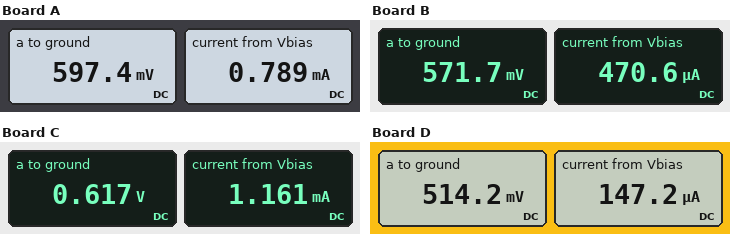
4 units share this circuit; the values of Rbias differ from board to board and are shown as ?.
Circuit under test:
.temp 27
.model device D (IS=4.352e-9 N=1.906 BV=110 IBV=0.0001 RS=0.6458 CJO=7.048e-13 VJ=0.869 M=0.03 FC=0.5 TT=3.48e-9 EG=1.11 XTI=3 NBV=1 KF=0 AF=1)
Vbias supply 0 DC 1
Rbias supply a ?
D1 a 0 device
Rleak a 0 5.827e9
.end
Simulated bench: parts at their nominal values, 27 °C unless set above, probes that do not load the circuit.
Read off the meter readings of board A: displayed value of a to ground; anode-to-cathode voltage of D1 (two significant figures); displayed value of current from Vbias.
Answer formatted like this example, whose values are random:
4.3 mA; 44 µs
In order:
597.4 mV; 600 mV; 0.789 mA
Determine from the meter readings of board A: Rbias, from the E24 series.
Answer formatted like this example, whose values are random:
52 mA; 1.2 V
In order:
510 Ω
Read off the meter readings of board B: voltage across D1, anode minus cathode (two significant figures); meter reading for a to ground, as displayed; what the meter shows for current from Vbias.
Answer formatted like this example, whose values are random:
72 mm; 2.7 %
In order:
570 mV; 571.7 mV; 470.6 µA
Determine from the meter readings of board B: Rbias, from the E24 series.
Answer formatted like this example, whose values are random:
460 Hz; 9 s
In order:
910 Ω
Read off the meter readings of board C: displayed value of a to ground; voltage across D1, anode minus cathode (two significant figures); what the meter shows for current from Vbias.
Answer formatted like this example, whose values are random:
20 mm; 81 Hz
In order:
0.617 V; 620 mV; 1.161 mA
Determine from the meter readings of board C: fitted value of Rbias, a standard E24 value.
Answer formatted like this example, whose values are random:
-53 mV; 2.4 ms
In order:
330 Ω
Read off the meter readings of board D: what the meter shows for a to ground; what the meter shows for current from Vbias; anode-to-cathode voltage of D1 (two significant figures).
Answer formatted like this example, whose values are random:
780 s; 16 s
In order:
514.2 mV; 147.2 µA; 510 mV
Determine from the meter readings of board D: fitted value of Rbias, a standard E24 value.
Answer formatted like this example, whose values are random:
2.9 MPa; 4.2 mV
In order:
3.3 kΩ
